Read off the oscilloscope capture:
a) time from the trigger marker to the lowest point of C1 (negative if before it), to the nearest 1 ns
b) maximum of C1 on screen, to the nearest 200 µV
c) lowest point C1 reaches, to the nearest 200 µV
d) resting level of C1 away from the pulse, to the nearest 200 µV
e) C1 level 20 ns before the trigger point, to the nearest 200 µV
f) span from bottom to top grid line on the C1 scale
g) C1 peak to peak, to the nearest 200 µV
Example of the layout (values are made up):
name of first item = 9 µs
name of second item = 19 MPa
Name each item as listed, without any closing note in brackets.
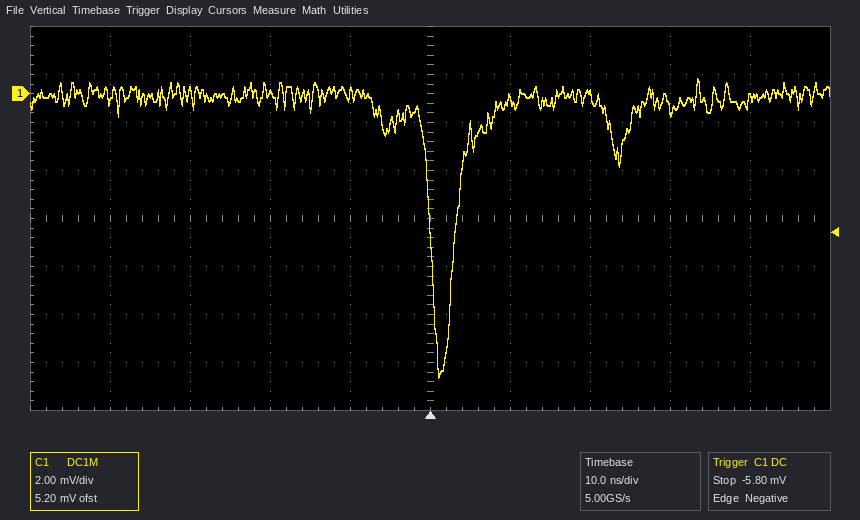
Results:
time from the trigger marker to the lowest point of C1 (negative if before it), to the nearest 1 ns = +1 ns
maximum of C1 on screen, to the nearest 200 µV = 600 µV
lowest point C1 reaches, to the nearest 200 µV = -11.8 mV
resting level of C1 away from the pulse, to the nearest 200 µV = -200 µV
C1 level 20 ns before the trigger point, to the nearest 200 µV = 0.0 mV
span from bottom to top grid line on the C1 scale = 16 mV
C1 peak to peak, to the nearest 200 µV = 12.4 mV
